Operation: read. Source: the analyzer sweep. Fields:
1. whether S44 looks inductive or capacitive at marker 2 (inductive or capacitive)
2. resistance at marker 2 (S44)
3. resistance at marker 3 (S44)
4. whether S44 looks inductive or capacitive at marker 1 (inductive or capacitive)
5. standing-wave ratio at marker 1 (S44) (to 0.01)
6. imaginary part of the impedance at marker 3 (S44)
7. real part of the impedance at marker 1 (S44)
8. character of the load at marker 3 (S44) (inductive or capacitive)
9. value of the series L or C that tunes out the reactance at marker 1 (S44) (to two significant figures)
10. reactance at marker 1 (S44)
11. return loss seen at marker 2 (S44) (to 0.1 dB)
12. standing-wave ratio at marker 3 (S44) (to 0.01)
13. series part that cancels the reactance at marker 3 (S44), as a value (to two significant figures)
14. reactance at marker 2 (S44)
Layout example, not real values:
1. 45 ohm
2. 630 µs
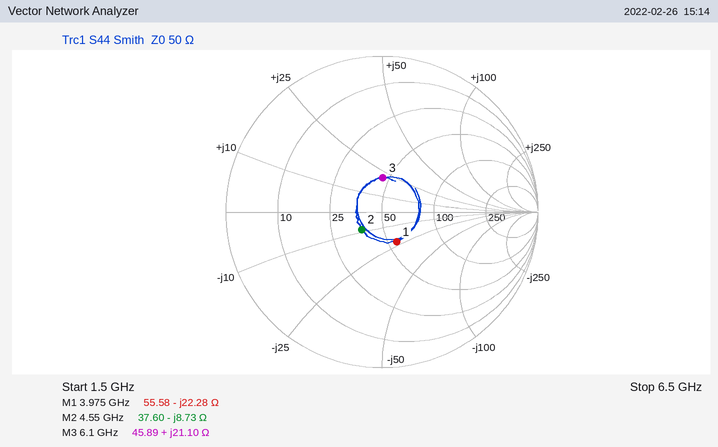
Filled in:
1. capacitive
2. 37.60 Ω
3. 45.89 Ω
4. capacitive
5. 1.54
6. +21.10 Ω
7. 55.58 Ω
8. inductive
9. 890 pH
10. -22.28 Ω
11. 15.3 dB
12. 1.56
13. 1.2 pF
14. -8.73 Ω
